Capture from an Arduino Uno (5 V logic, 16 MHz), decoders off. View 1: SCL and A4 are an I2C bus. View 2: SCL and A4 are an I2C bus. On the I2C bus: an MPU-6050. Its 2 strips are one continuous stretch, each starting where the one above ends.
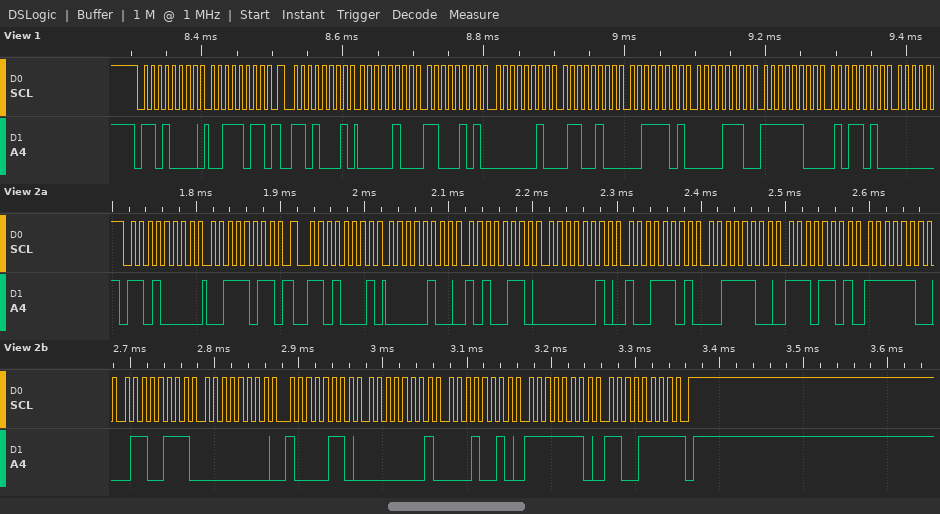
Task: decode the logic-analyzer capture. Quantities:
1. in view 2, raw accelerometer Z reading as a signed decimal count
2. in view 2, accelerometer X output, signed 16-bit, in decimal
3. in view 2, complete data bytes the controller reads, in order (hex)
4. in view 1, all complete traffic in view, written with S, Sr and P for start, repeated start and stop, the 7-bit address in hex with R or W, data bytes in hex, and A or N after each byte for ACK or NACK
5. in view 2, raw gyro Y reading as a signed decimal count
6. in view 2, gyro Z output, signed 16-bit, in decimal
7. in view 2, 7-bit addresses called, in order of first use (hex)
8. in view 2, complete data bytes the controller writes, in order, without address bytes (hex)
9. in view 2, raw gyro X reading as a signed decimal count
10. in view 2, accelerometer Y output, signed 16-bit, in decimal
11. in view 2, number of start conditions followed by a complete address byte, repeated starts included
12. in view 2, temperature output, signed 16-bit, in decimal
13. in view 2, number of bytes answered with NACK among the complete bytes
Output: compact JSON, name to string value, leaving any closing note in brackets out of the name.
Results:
{"in view 2, raw accelerometer Z reading as a signed decimal count": "15597", "in view 2, accelerometer X output, signed 16-bit, in decimal": "1190", "in view 2, complete data bytes the controller reads, in order": "04 A6 02 9D 3C ED FC 67 00 86 01 12 FE CF", "in view 1, all complete traffic in view, written with S, Sr and P for start, repeated start and stop, the 7-bit address in hex with R or W, data bytes in hex, and A or N after each byte for ACK or NACK": "S 68W A 3B A Sr 68R A 04 A C5 A 02 A 64 A 3D A 0E A FC A 5A A", "in view 2, raw gyro Y reading as a signed decimal count": "274", "in view 2, gyro Z output, signed 16-bit, in decimal": "-305", "in view 2, 7-bit addresses called, in order of first use": "0x68", "in view 2, complete data bytes the controller writes, in order, without address bytes": "3B", "in view 2, raw gyro X reading as a signed decimal count": "134", "in view 2, accelerometer Y output, signed 16-bit, in decimal": "669", "in view 2, number of start conditions followed by a complete address byte, repeated starts included": "2", "in view 2, temperature output, signed 16-bit, in decimal": "-921", "in view 2, number of bytes answered with NACK among the complete bytes": "1"}
